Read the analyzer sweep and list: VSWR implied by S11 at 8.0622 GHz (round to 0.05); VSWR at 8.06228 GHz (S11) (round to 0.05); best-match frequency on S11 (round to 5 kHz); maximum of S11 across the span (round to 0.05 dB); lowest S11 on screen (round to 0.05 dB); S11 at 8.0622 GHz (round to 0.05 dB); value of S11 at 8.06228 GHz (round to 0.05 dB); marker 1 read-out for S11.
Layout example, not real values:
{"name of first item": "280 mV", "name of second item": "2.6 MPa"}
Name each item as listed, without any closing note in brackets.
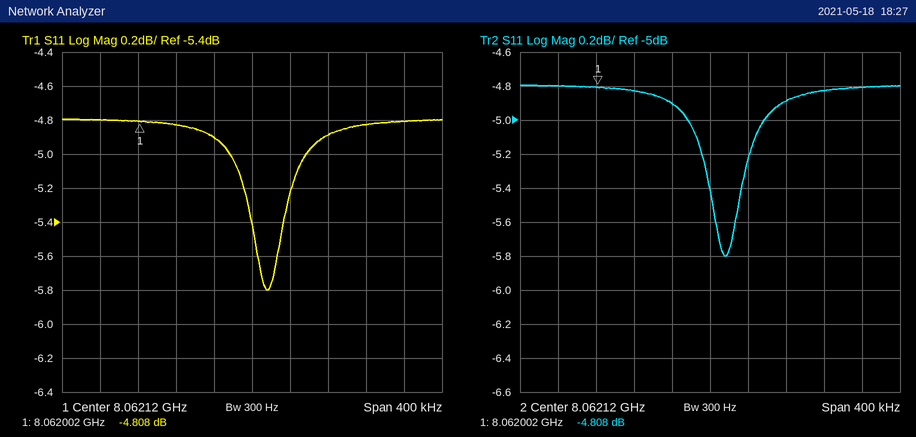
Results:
{"VSWR implied by S11 at 8.0622 GHz": "3.65", "VSWR at 8.06228 GHz (S11)": "3.70", "best-match frequency on S11": "8.062135 GHz", "maximum of S11 across the span": "-4.80 dB", "lowest S11 on screen": "-5.80 dB", "S11 at 8.0622 GHz": "-4.90 dB", "value of S11 at 8.06228 GHz": "-4.80 dB", "marker 1 read-out for S11": "-4.808 dB"}
